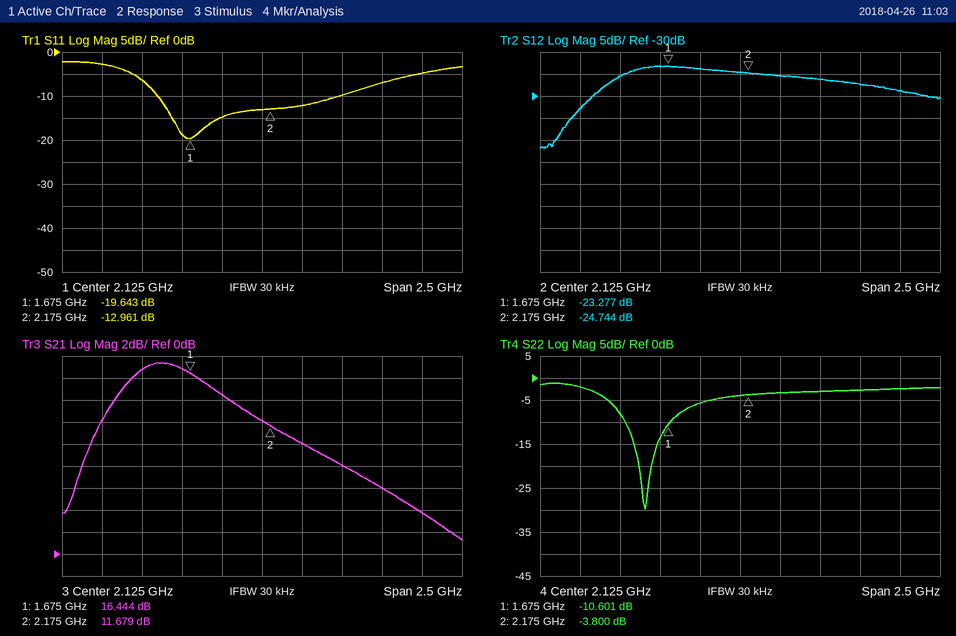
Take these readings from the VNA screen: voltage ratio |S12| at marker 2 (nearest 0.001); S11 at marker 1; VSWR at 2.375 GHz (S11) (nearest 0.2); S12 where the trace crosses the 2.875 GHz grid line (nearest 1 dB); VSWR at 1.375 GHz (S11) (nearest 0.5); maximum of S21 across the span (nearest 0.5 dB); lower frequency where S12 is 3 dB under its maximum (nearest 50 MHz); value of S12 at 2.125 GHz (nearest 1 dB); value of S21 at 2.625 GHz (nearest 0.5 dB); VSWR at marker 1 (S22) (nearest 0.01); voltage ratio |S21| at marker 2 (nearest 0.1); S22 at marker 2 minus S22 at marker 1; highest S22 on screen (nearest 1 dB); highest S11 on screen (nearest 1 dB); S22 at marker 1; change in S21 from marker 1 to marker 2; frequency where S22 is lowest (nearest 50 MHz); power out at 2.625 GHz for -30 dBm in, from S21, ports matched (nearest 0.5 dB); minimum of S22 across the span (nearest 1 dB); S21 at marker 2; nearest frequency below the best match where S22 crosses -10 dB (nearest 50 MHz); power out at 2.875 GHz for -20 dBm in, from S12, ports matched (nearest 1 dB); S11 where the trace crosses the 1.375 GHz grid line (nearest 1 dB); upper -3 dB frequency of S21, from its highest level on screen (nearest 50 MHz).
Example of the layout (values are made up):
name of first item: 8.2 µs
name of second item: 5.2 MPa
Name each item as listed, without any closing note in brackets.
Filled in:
voltage ratio |S12| at marker 2: 0.058
S11 at marker 1: -19.643 dB
VSWR at 2.375 GHz (S11): 1.6
S12 where the trace crosses the 2.875 GHz grid line: -27 dB
VSWR at 1.375 GHz (S11): 3.0
maximum of S21 across the span: 17.5 dB
lower frequency where S12 is 3 dB under its maximum: 1.35 GHz
value of S12 at 2.125 GHz: -25 dB
value of S21 at 2.625 GHz: 8.0 dB
VSWR at marker 1 (S22): 1.84
voltage ratio |S21| at marker 2: 3.8
S22 at marker 2 minus S22 at marker 1: 6.801 dB
highest S22 on screen: -1 dB
highest S11 on screen: -2 dB
S22 at marker 1: -10.601 dB
change in S21 from marker 1 to marker 2: -4.765 dB
frequency where S22 is lowest: 1.55 GHz
power out at 2.625 GHz for -30 dBm in, from S21, ports matched: -22.0 dBm
minimum of S22 across the span: -30 dB
S21 at marker 2: 11.679 dB
nearest frequency below the best match where S22 crosses -10 dB: 1.40 GHz
power out at 2.875 GHz for -20 dBm in, from S12, ports matched: -47 dBm
S11 where the trace crosses the 1.375 GHz grid line: -6 dB
upper -3 dB frequency of S21, from its highest level on screen: 1.90 GHz
